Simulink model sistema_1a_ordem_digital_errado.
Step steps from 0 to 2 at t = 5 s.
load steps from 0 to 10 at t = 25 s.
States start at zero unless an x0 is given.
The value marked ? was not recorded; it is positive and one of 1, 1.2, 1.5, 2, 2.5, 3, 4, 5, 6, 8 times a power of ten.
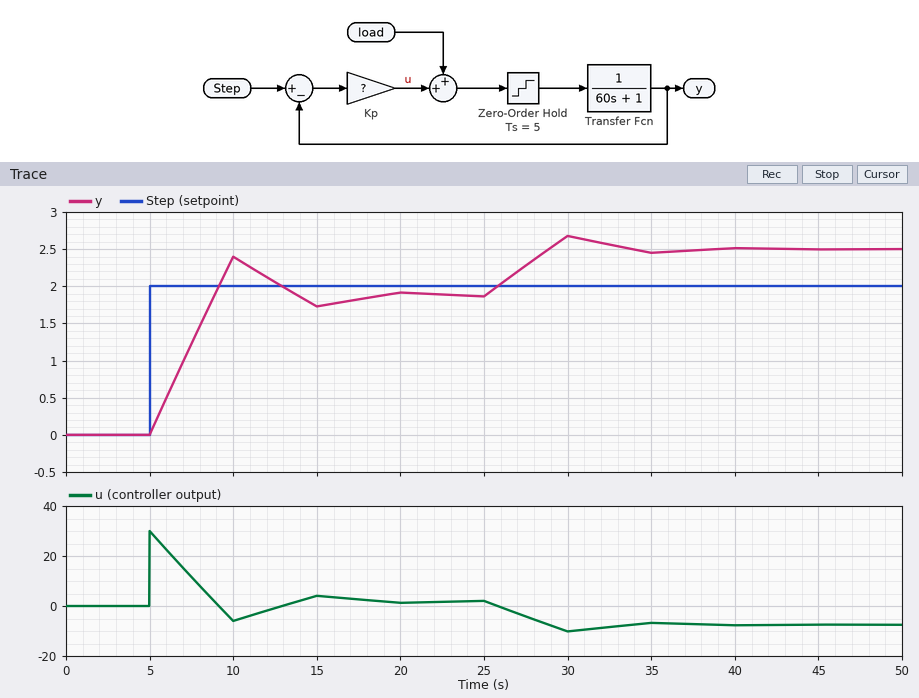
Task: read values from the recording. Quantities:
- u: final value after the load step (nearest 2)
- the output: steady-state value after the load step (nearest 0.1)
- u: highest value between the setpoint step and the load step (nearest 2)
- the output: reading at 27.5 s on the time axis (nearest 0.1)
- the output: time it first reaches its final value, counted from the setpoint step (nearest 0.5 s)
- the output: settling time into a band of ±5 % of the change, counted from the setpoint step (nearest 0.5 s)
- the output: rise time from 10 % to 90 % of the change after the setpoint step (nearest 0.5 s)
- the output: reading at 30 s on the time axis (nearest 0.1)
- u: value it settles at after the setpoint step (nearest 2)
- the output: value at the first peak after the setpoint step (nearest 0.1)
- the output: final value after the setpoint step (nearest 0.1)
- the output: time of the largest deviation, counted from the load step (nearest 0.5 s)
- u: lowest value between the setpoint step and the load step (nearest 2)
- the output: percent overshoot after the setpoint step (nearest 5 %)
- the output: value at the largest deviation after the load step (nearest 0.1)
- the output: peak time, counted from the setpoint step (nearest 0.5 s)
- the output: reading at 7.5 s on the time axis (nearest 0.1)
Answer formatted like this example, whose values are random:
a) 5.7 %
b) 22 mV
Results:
a) -8
b) 2.5
c) 30
d) 2.3
e) 4.0 s
f) 11.5 s
g) 3.0 s
h) 2.7
i) 2
j) 2.4
k) 1.9
l) 5.0 s
m) -6
n) 30 %
o) 2.7
p) 5.0 s
q) 1.2
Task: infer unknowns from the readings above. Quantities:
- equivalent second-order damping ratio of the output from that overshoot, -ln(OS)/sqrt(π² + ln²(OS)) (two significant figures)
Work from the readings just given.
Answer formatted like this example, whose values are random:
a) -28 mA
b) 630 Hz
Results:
a) 0.36
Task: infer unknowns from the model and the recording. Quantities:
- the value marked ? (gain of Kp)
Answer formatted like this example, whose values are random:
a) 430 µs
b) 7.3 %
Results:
a) 15
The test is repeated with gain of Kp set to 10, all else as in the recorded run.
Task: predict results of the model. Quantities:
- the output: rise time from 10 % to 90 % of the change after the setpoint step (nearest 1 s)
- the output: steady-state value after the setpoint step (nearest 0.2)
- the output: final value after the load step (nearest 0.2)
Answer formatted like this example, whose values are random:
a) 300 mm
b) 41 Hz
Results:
a) 5 s
b) 1.8
c) 2.8
